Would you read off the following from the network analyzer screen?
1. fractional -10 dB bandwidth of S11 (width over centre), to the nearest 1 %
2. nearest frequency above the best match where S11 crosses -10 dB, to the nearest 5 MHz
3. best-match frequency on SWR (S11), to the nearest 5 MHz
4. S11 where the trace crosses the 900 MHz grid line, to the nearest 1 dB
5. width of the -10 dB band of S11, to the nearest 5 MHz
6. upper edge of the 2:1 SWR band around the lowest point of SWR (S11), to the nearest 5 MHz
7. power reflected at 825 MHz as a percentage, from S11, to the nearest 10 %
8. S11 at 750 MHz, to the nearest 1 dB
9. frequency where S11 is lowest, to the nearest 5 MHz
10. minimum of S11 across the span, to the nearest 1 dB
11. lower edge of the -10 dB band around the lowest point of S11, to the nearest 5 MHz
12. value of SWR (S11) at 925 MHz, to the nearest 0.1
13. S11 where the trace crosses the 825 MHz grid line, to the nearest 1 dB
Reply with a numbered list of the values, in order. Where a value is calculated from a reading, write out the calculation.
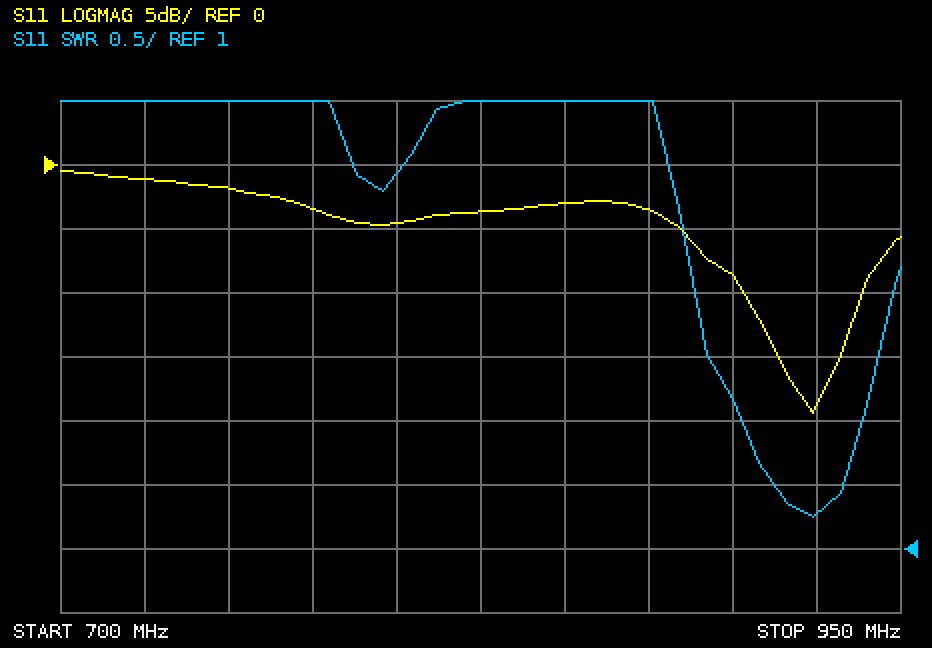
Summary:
1. 35 MHz / 922.5 MHz ≈ 4 %
2. 940 MHz
3. 925 MHz
4. -9 dB
5. 940 MHz − 905 MHz = 35 MHz
6. 940 MHz
7. 10^(-4/10) ≈ 40 %
8. -2 dB
9. 925 MHz
10. -19 dB
11. 905 MHz
12. 1.3
13. -4 dB
